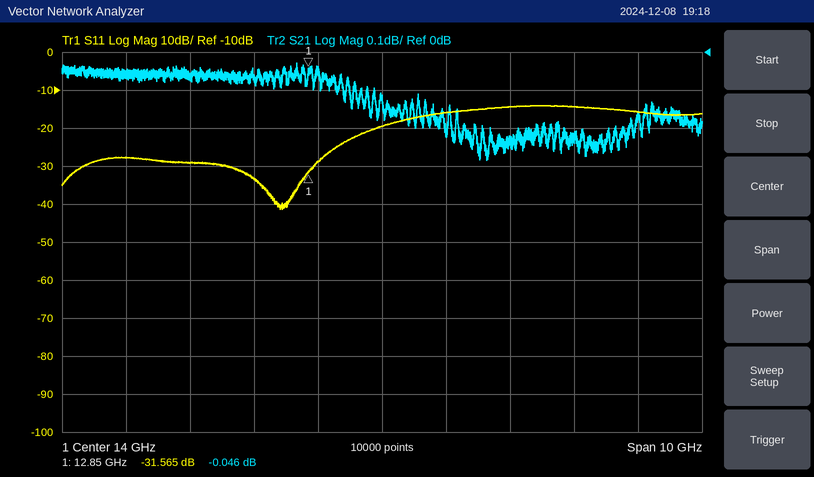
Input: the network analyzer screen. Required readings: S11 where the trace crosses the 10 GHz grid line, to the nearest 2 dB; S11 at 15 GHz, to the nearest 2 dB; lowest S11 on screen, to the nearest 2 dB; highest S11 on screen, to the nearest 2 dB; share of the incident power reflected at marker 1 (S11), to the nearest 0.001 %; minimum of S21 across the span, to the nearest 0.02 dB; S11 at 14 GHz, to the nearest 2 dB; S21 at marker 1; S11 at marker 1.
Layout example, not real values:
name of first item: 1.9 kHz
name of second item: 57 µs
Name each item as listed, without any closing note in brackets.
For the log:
S11 where the trace crosses the 10 GHz grid line, to the nearest 2 dB: -28 dB
S11 at 15 GHz, to the nearest 2 dB: -16 dB
lowest S11 on screen, to the nearest 2 dB: -42 dB
highest S11 on screen, to the nearest 2 dB: -14 dB
share of the incident power reflected at marker 1 (S11), to the nearest 0.001 %: 0.070 %
minimum of S21 across the span, to the nearest 0.02 dB: -0.28 dB
S11 at 14 GHz, to the nearest 2 dB: -20 dB
S21 at marker 1: -0.046 dB
S11 at marker 1: -31.565 dB
